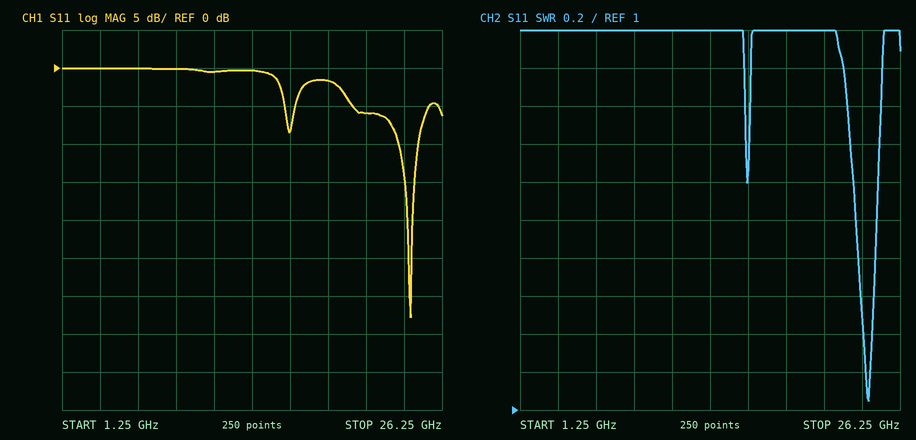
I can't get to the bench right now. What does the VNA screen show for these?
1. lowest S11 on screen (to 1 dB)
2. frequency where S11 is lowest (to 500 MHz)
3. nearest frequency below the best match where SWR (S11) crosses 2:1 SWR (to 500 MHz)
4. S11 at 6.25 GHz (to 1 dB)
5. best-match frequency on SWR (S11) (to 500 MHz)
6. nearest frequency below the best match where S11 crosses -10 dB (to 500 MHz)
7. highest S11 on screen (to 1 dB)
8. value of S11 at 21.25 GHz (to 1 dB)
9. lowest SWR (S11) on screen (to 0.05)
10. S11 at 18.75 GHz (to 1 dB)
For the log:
-33 dB
24.0 GHz
23.5 GHz
0 dB
24.0 GHz
23.5 GHz
0 dB
-6 dB
1.05
-2 dB
